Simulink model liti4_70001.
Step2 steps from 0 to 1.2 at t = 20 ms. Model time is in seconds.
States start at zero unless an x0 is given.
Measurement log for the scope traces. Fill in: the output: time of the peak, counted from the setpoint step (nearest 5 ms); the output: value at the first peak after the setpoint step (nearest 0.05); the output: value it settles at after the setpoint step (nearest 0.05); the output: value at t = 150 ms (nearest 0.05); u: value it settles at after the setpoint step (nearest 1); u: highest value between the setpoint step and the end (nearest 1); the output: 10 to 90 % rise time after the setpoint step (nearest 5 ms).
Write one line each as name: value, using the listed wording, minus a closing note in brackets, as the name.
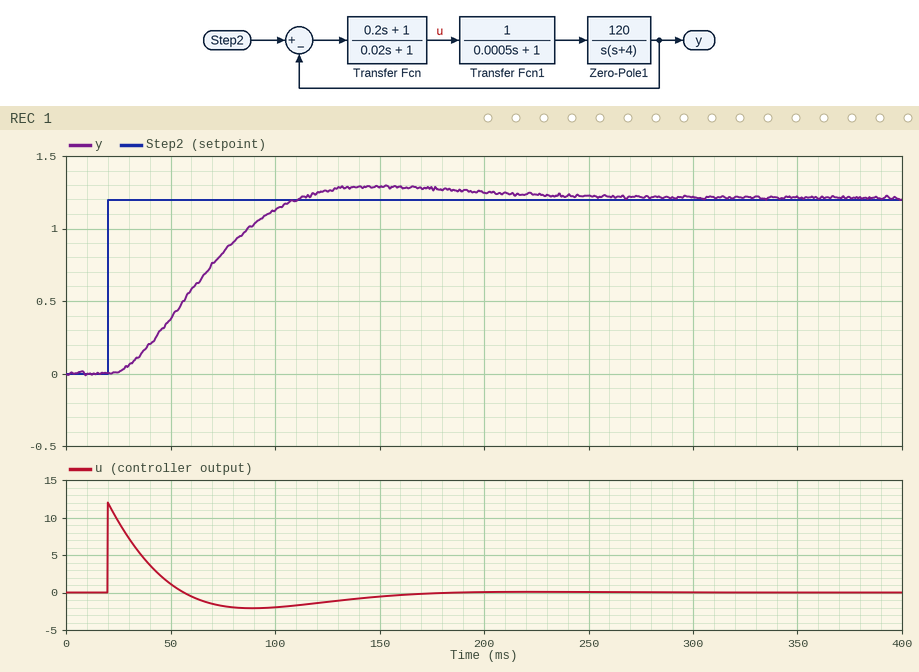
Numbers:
the output: time of the peak, counted from the setpoint step: 130 ms
the output: value at the first peak after the setpoint step: 1.30
the output: value it settles at after the setpoint step: 1.20
the output: value at t = 150 ms: 1.30
u: value it settles at after the setpoint step: 0
u: highest value between the setpoint step and the end: 12
the output: 10 to 90 % rise time after the setpoint step: 60 ms
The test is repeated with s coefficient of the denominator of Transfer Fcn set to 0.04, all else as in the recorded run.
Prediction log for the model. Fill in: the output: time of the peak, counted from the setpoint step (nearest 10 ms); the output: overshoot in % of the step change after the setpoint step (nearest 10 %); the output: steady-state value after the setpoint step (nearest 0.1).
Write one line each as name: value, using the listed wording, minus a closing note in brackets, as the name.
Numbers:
the output: time of the peak, counted from the setpoint step: 150 ms
the output: overshoot in % of the step change after the setpoint step: 20 %
the output: steady-state value after the setpoint step: 1.2
